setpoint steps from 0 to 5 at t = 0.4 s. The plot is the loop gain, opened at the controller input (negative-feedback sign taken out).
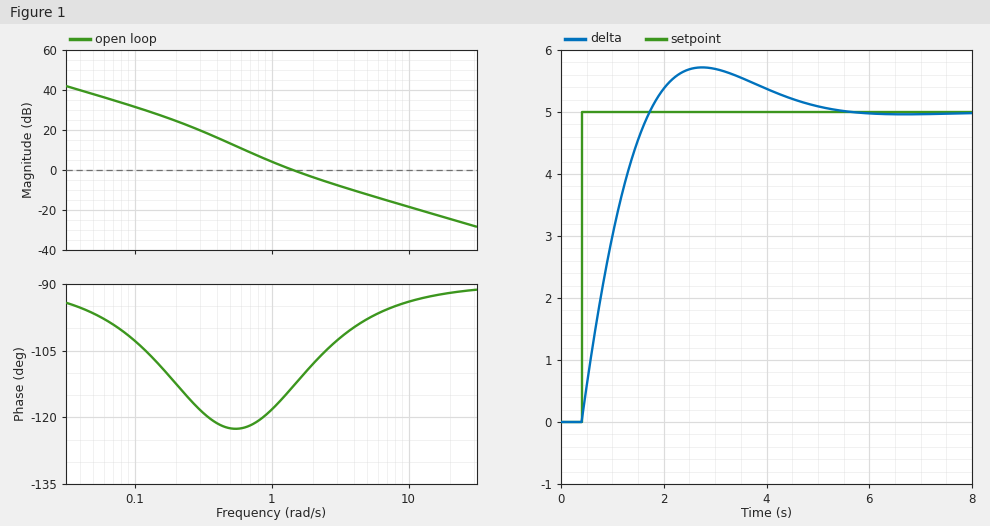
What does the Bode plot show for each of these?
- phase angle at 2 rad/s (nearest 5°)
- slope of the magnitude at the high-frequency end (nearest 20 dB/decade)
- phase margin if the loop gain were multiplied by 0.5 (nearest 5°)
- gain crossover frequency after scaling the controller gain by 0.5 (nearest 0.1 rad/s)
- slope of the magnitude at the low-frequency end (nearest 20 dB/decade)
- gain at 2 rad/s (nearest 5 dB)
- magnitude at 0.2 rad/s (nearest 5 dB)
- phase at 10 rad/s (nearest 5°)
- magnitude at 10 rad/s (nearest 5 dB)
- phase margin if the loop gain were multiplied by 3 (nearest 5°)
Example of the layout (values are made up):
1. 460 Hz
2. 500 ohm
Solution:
1. -110°
2. -20 dB/decade
3. 60°
4. 0.9 rad/s
5. -20 dB/decade
6. -5 dB
7. 25 dB
8. -95°
9. -20 dB
10. 80°
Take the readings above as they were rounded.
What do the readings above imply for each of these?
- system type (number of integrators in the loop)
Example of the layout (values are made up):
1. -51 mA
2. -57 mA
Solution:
1. 1
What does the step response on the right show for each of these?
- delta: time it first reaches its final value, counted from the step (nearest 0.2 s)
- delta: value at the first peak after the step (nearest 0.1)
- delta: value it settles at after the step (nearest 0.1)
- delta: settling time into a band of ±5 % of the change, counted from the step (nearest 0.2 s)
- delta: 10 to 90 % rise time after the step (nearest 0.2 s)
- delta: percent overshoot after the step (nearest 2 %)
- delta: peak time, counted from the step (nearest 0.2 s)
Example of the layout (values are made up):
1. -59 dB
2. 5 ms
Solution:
1. 1.4 s
2. 5.7
3. 5.0
4. 4.0 s
5. 1.0 s
6. 14 %
7. 2.4 s
